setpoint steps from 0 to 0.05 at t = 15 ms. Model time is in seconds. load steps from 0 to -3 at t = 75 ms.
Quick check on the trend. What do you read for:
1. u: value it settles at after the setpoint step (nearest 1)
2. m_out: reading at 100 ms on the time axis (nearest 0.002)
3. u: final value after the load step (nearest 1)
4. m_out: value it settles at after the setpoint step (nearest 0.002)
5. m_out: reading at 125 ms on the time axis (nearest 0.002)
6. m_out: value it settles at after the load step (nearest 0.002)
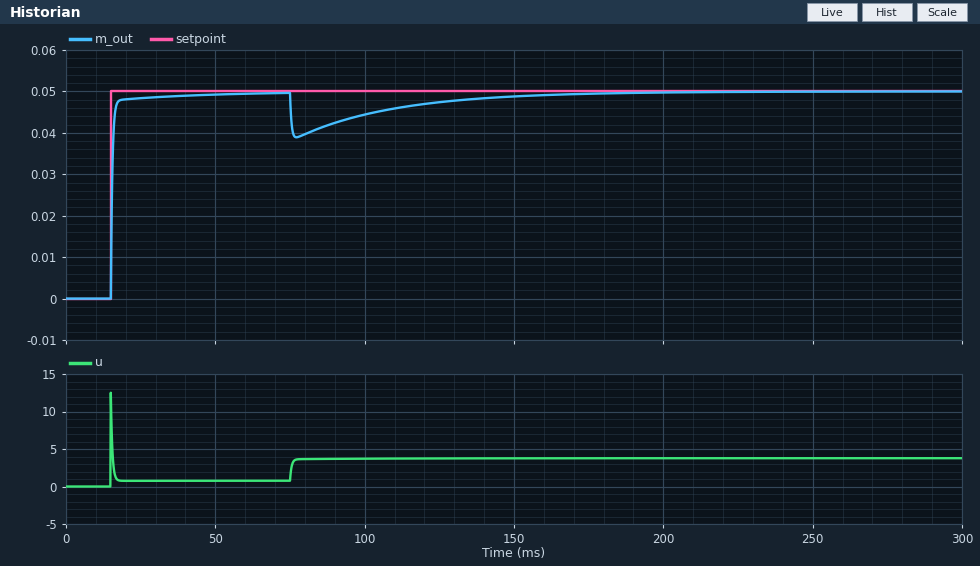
1
0.044
4
0.050
0.048
0.050
